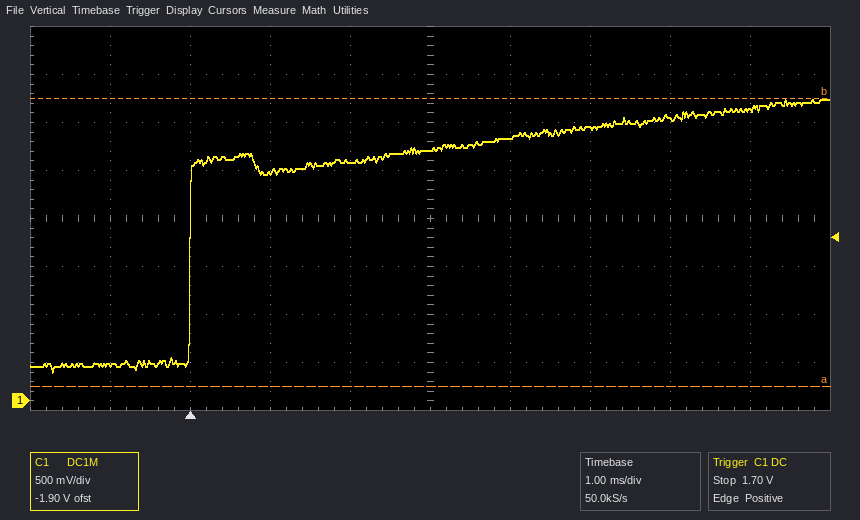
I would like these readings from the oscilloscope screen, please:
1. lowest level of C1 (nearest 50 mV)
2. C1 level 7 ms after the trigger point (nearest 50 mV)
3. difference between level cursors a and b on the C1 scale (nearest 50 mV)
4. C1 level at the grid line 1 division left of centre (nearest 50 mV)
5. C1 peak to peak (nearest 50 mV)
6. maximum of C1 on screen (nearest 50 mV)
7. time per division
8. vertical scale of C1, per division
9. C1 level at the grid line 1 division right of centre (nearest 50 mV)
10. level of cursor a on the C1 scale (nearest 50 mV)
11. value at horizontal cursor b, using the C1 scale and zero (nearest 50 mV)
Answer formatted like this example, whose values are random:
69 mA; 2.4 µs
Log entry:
300 mV; 3.05 V; 3.00 V; 2.50 V; 2.85 V; 3.15 V; 1 ms; 500 mV; 2.75 V; 150 mV; 3.15 V
